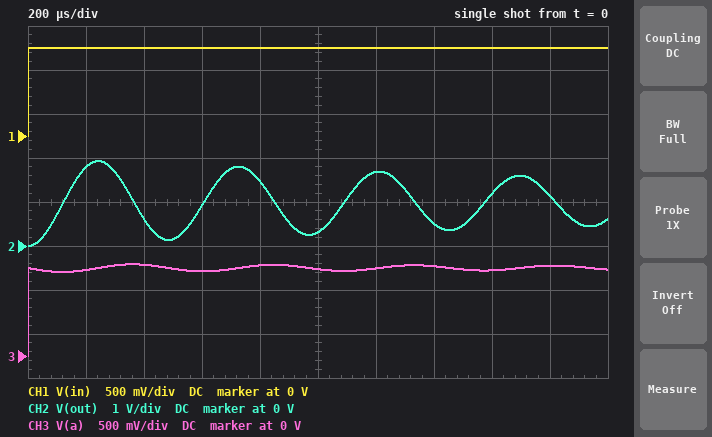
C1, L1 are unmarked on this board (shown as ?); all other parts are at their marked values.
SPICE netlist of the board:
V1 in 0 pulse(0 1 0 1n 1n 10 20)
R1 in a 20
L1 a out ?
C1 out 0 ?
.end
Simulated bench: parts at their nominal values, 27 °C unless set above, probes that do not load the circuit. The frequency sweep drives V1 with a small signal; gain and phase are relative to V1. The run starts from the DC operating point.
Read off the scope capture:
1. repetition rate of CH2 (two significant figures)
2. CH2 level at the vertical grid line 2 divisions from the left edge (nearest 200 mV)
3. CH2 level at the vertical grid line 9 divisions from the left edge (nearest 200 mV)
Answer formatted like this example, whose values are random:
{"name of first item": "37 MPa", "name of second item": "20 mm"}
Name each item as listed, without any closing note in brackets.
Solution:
{"repetition rate of CH2": "2.1 kHz", "CH2 level at the vertical grid line 2 divisions from the left edge": "600 mV", "CH2 level at the vertical grid line 9 divisions from the left edge": "1.2 V"}
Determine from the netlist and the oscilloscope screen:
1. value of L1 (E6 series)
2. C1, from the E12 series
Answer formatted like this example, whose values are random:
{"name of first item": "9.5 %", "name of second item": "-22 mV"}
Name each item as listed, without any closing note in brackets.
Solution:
{"value of L1": "33 mH", "C1, from the E12 series": "180 nF"}
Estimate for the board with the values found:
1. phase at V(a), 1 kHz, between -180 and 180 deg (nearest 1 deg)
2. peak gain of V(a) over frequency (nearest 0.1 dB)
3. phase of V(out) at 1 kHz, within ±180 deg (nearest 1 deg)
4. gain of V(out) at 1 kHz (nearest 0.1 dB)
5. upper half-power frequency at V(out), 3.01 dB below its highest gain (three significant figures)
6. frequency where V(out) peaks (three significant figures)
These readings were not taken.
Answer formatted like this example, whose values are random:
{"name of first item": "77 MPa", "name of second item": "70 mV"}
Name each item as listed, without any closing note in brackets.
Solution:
{"phase at V(a), 1 kHz, between -180 and 180 deg": "-2 deg", "peak gain of V(a) over frequency": "0 dB", "phase of V(out) at 1 kHz, within ±180 deg": "-2 deg", "gain of V(out) at 1 kHz": "2.3 dB", "upper half-power frequency at V(out), 3.01 dB below its highest gain": "2.11 kHz", "frequency where V(out) peaks": "2.06 kHz"}
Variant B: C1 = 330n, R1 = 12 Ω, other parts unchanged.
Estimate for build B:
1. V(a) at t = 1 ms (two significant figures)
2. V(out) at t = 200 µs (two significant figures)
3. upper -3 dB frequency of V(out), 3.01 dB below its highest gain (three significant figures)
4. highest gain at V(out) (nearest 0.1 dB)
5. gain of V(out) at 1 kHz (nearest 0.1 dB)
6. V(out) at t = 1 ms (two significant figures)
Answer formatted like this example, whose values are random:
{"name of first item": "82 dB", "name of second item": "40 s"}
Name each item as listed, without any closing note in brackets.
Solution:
{"V(a) at t = 1 ms": "1.0 V", "V(out) at t = 200 µs": "1.3 V", "upper -3 dB frequency of V(out), 3.01 dB below its highest gain": "1.55 kHz", "highest gain at V(out)": "28.4 dB", "gain of V(out) at 1 kHz": "4.9 dB", "V(out) at t = 1 ms": "1.8 V"}
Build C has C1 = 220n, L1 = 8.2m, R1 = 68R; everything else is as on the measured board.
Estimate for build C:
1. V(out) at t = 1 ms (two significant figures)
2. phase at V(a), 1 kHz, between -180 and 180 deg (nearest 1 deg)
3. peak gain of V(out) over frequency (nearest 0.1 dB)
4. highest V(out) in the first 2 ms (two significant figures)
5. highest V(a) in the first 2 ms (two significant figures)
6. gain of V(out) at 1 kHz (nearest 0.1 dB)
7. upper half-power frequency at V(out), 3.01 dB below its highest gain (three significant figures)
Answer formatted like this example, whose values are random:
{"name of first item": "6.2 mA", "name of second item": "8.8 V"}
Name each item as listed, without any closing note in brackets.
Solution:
{"V(out) at t = 1 ms": "1.0 V", "phase at V(a), 1 kHz, between -180 and 180 deg": "-6 deg", "peak gain of V(out) over frequency": "9.2 dB", "highest V(out) in the first 2 ms": "1.6 V", "highest V(a) in the first 2 ms": "1.2 V", "gain of V(out) at 1 kHz": "0.6 dB", "upper half-power frequency at V(out), 3.01 dB below its highest gain": "4.25 kHz"}
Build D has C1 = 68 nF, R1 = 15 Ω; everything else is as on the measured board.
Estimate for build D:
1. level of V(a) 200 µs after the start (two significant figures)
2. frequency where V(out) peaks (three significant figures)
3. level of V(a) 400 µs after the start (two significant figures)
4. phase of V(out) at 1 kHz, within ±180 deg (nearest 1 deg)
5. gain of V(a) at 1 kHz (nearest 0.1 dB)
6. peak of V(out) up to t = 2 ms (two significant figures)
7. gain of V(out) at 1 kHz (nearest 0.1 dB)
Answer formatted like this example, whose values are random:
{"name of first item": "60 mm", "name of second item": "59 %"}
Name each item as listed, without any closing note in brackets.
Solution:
{"level of V(a) 200 µs after the start": "1.0 V", "frequency where V(out) peaks": "3.36 kHz", "level of V(a) 400 µs after the start": "980 mV", "phase of V(out) at 1 kHz, within ±180 deg": "0 deg", "gain of V(a) at 1 kHz": "0 dB", "peak of V(out) up to t = 2 ms": "2.0 V", "gain of V(out) at 1 kHz": "0.8 dB"}
